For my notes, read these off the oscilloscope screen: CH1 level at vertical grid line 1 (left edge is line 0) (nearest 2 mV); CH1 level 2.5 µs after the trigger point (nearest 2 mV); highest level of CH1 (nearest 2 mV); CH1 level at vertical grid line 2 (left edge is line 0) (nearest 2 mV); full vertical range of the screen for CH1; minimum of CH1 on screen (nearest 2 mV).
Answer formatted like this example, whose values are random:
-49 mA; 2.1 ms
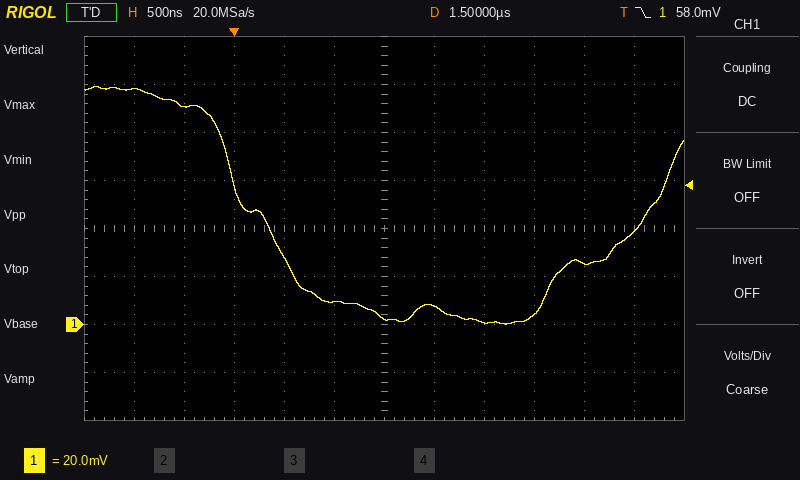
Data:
98 mV; 0 mV; 100 mV; 90 mV; 160 mV; 0 mV
